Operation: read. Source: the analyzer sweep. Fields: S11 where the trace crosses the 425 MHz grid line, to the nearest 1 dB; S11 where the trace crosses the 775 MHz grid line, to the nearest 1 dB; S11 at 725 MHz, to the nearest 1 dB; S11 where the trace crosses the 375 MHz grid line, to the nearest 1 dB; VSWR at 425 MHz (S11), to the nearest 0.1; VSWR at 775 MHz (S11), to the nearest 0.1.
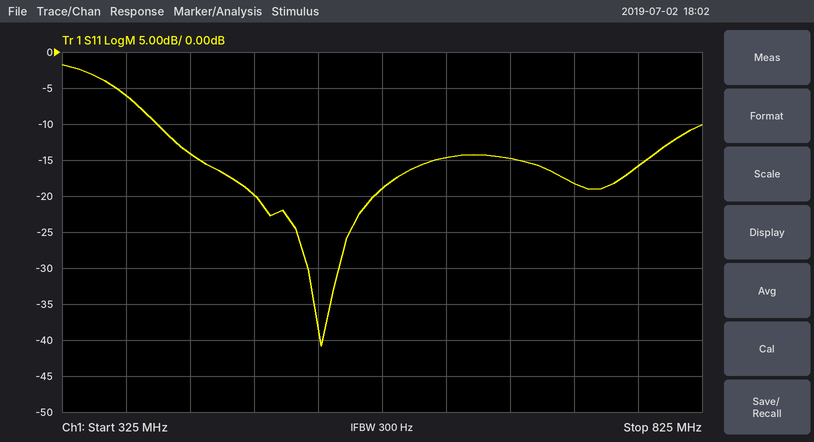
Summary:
-14 dB
-16 dB
-18 dB
-6 dB
1.5
1.4
